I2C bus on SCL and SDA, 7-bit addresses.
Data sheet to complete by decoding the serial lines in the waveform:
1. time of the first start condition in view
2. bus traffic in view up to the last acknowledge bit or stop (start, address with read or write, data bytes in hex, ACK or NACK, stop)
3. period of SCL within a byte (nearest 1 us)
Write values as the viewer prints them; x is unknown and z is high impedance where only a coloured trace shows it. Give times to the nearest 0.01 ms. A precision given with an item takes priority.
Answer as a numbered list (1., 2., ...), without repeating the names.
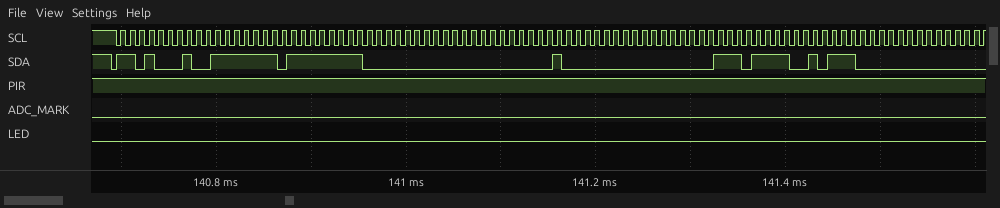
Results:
1. 140.69 ms
2. start, address 68 read ACK, 7F ACK, FF ACK, 00 ACK, 00 ACK, 40 ACK, 00 ACK, EF ACK, 5C ACK, 00 ACK
3. 10 us
